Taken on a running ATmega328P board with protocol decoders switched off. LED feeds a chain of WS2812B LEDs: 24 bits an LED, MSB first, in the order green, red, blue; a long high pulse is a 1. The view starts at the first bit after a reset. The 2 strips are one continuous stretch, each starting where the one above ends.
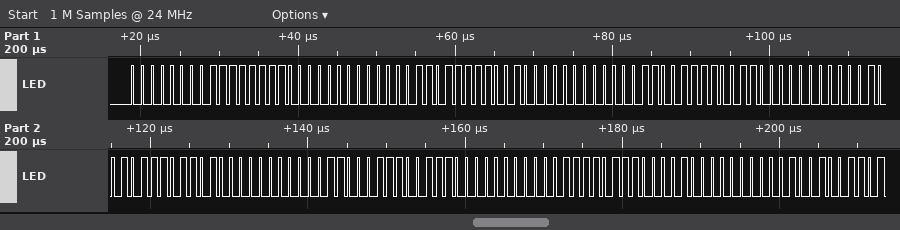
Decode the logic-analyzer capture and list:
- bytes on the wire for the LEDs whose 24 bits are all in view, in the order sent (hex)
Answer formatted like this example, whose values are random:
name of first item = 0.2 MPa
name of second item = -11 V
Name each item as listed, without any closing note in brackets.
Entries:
bytes on the wire for the LEDs whose 24 bits are all in view, in the order sent = 00 FF 00 06 F9 00 0C F3 00 12 ED 00 18 E7 00 1E E1 00
